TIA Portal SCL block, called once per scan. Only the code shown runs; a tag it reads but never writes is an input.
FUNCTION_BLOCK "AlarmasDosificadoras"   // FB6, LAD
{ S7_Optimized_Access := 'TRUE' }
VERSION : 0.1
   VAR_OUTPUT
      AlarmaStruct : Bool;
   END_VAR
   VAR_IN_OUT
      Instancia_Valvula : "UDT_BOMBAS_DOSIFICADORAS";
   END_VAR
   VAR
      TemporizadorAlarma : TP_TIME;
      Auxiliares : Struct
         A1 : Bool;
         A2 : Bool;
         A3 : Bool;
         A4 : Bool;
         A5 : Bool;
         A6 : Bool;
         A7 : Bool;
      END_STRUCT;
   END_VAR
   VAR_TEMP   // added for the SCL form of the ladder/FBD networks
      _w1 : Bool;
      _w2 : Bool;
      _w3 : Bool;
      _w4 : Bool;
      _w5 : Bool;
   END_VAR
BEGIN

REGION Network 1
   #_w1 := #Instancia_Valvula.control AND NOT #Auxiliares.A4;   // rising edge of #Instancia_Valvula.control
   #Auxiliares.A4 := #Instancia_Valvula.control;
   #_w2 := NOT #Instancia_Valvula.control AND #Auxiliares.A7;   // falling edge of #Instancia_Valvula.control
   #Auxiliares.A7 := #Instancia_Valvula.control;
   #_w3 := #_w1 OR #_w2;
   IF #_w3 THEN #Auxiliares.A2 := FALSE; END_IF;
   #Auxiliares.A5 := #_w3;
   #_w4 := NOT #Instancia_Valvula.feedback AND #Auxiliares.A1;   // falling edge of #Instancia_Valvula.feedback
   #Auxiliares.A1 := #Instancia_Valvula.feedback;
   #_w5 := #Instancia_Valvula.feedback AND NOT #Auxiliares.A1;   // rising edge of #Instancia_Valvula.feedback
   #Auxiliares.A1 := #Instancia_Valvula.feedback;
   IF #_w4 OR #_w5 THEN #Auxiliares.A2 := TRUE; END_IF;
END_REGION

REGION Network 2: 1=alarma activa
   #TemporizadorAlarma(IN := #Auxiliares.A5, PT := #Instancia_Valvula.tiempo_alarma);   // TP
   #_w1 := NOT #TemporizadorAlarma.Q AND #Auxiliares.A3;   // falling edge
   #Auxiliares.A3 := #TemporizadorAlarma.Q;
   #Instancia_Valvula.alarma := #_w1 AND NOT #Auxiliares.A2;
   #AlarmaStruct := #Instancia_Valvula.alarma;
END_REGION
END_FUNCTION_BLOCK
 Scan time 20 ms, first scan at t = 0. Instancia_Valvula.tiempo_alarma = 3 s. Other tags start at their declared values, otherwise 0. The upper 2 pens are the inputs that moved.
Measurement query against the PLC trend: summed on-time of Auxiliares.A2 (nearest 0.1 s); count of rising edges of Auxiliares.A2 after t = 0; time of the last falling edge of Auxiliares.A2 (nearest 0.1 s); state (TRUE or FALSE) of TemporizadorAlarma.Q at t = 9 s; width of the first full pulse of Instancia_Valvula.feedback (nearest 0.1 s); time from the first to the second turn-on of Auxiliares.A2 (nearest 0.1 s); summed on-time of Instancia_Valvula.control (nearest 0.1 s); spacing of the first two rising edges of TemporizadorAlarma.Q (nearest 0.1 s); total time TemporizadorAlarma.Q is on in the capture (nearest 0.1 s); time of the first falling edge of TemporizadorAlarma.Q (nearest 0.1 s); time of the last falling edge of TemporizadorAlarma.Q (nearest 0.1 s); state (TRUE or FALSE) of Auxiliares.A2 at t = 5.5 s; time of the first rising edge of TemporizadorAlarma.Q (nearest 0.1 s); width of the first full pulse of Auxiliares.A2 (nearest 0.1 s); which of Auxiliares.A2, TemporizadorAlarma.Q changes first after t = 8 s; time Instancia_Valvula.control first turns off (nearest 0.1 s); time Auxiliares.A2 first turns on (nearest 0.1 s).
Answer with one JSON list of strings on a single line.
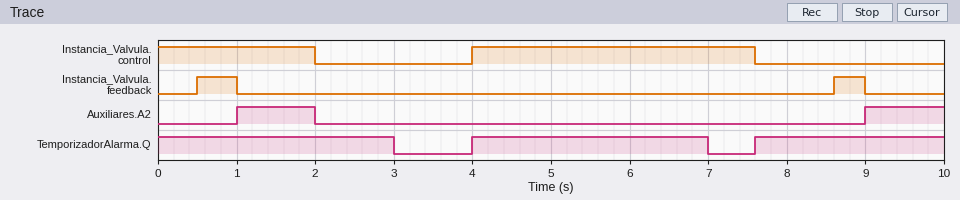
["2.0 s", "2", "2.0 s", "TRUE", "0.5 s", "8.0 s", "5.6 s", "3.6 s", "8.4 s", "3.0 s", "7.0 s", "FALSE", "4.0 s", "1.0 s", "Auxiliares.A2", "2.0 s", "1.0 s"]
